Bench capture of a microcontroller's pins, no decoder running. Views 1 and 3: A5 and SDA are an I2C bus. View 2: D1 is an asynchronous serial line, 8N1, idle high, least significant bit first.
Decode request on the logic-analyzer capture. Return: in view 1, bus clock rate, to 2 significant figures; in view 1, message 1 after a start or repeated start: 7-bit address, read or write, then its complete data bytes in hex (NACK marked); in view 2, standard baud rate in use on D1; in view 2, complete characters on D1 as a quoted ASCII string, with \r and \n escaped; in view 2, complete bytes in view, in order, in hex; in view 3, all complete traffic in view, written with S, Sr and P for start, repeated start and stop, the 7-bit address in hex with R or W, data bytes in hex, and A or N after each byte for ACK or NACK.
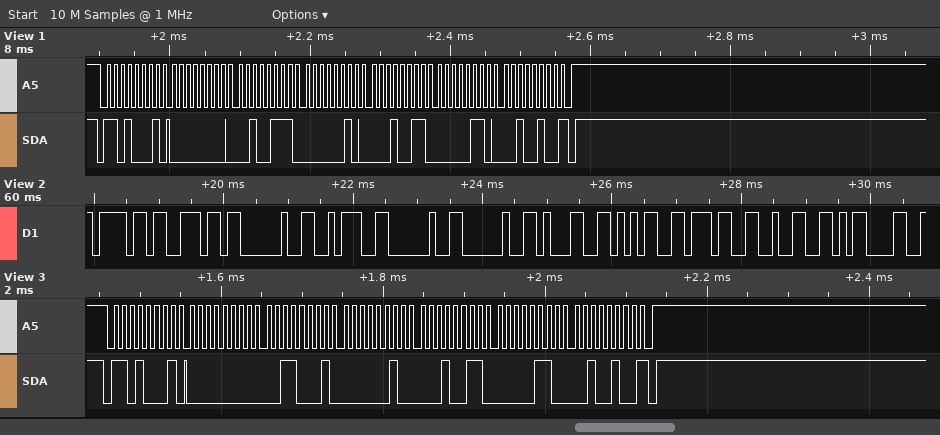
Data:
100 kHz
0x68 read: 00 27 02 13 06 24 NACK
9600 baud
"on :  1572\r"
0x6F 0x6E 0x20 0x3A 0x20 0x20 0x31 0x35 0x37 0x32 0x0D
S 68R A 00 A 31 A 02 A 13 A 06 A 24 N P
